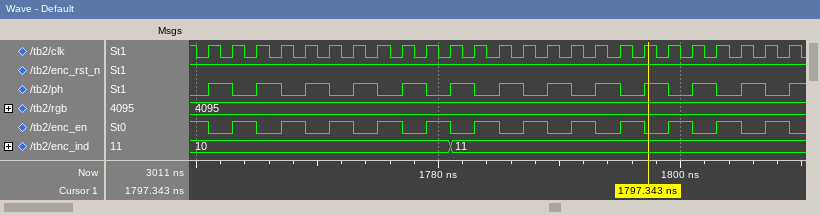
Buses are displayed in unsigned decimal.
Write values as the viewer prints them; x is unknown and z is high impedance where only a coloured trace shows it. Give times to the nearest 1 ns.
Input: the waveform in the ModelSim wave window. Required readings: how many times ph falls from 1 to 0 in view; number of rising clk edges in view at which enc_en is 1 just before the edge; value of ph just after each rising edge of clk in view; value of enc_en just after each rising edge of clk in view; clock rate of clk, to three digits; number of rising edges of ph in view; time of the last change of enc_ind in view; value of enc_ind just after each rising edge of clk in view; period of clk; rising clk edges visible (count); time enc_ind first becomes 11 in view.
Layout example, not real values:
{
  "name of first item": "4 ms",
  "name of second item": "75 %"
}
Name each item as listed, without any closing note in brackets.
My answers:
{
  "how many times ph falls from 1 to 0 in view": "12",
  "number of rising clk edges in view at which enc_en is 1 just before the edge": "13",
  "value of ph just after each rising edge of clk in view": "1 0 1 0 1 0 1 0 1 0 1 0 1 0 1 0 1 0 1 0 1 0 1 0 1",
  "value of enc_en just after each rising edge of clk in view": "0 1 0 1 0 1 0 1 0 1 0 1 0 1 0 1 0 1 0 1 0 1 0 1 0",
  "clock rate of clk, to three digits": "500 MHz",
  "number of rising edges of ph in view": "13",
  "time of the last change of enc_ind in view": "1781 ns",
  "value of enc_ind just after each rising edge of clk in view": "10, 10, 10, 10, 10, 10, 10, 10, 10, 10, 11, 11, 11, 11, 11, 11, 11, 11, 11, 11, 11, 11, 11, 11, 11",
  "period of clk": "2 ns",
  "rising clk edges visible": "25",
  "time enc_ind first becomes 11 in view": "1781 ns"
}
